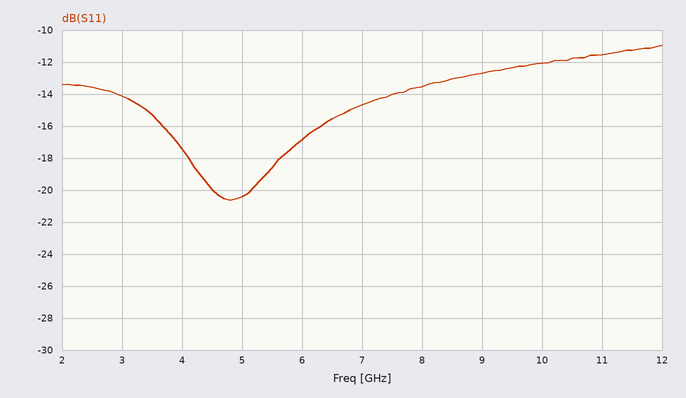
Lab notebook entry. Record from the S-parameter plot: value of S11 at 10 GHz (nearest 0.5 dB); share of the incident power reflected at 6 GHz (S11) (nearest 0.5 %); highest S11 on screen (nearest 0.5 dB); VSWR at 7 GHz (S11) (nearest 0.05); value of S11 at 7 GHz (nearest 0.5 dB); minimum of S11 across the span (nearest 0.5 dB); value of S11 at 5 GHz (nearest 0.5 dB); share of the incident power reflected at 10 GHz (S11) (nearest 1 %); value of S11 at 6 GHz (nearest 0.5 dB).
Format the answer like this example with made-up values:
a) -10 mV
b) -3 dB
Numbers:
a) -12.0 dB
b) 2.0 %
c) -11.0 dB
d) 1.45
e) -14.5 dB
f) -20.5 dB
g) -20.5 dB
h) 6 %
i) -17.0 dB
